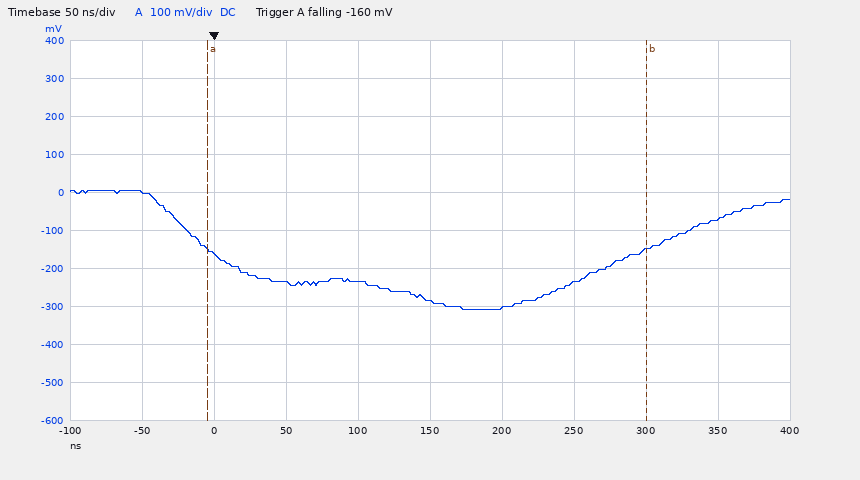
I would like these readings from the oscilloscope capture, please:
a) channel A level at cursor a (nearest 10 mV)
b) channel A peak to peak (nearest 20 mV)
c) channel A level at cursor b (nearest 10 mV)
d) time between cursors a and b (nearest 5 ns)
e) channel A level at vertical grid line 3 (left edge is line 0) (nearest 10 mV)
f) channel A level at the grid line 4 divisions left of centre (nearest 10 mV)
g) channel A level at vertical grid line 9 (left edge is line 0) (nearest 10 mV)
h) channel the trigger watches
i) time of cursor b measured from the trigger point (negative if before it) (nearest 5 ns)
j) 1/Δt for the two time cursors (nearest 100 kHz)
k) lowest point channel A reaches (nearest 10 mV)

-150 mV
320 mV
-150 mV
305 ns
-240 mV
0 mV
-70 mV
channel A
+300 ns
3.3 MHz
-310 mV
